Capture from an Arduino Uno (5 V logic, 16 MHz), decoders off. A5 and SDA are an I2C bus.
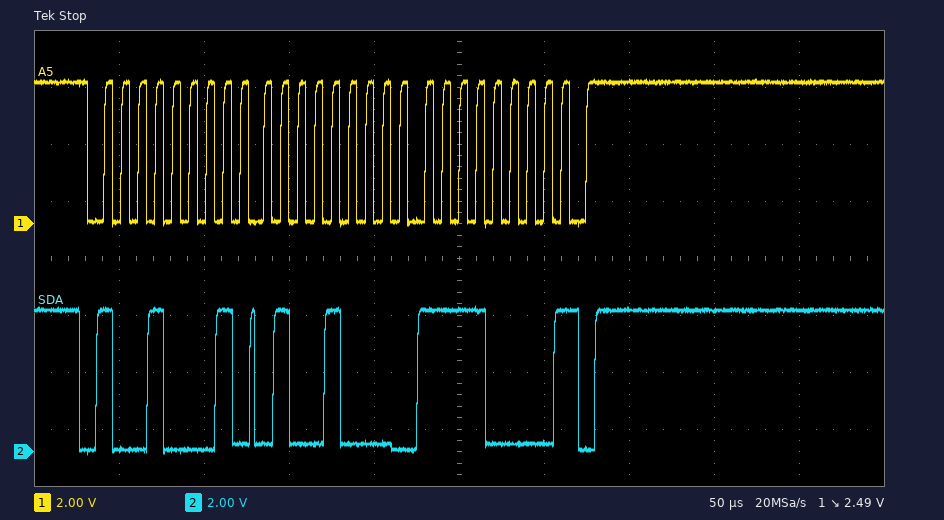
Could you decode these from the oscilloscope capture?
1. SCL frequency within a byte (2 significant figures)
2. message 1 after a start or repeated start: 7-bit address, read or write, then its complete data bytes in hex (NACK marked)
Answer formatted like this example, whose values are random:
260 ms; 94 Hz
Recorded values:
100 kHz; 0x48 read: 48 F0 NACK
